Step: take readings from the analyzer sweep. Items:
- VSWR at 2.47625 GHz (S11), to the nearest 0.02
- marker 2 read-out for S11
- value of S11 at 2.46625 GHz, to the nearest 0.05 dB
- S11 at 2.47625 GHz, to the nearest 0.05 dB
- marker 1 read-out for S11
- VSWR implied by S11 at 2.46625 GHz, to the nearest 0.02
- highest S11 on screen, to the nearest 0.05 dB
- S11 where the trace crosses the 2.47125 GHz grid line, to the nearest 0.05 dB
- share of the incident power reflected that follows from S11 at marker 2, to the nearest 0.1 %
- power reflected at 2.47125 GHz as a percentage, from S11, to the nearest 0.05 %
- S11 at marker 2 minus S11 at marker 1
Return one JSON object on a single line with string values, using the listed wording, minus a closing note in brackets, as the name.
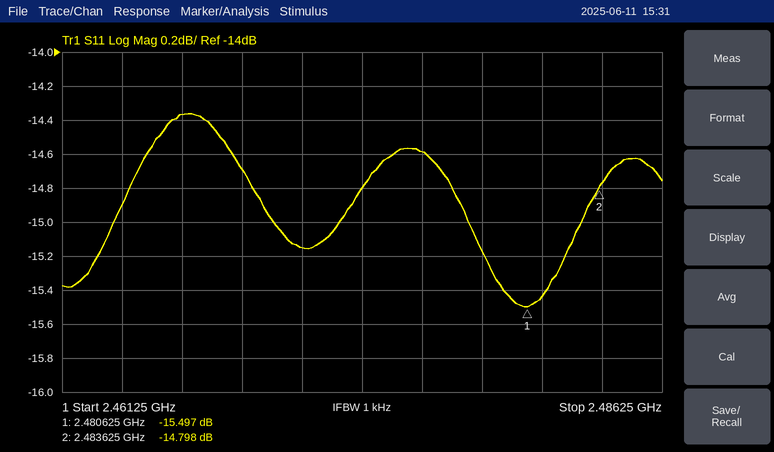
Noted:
{"VSWR at 2.47625 GHz (S11), to the nearest 0.02": "1.46", "marker 2 read-out for S11": "-14.798 dB", "value of S11 at 2.46625 GHz, to the nearest 0.05 dB": "-14.35 dB", "S11 at 2.47625 GHz, to the nearest 0.05 dB": "-14.60 dB", "marker 1 read-out for S11": "-15.497 dB", "VSWR implied by S11 at 2.46625 GHz, to the nearest 0.02": "1.48", "highest S11 on screen, to the nearest 0.05 dB": "-14.35 dB", "S11 where the trace crosses the 2.47125 GHz grid line, to the nearest 0.05 dB": "-15.15 dB", "share of the incident power reflected that follows from S11 at marker 2, to the nearest 0.1 %": "3.3 %", "power reflected at 2.47125 GHz as a percentage, from S11, to the nearest 0.05 %": "3.05 %", "S11 at marker 2 minus S11 at marker 1": "0.699 dB"}
